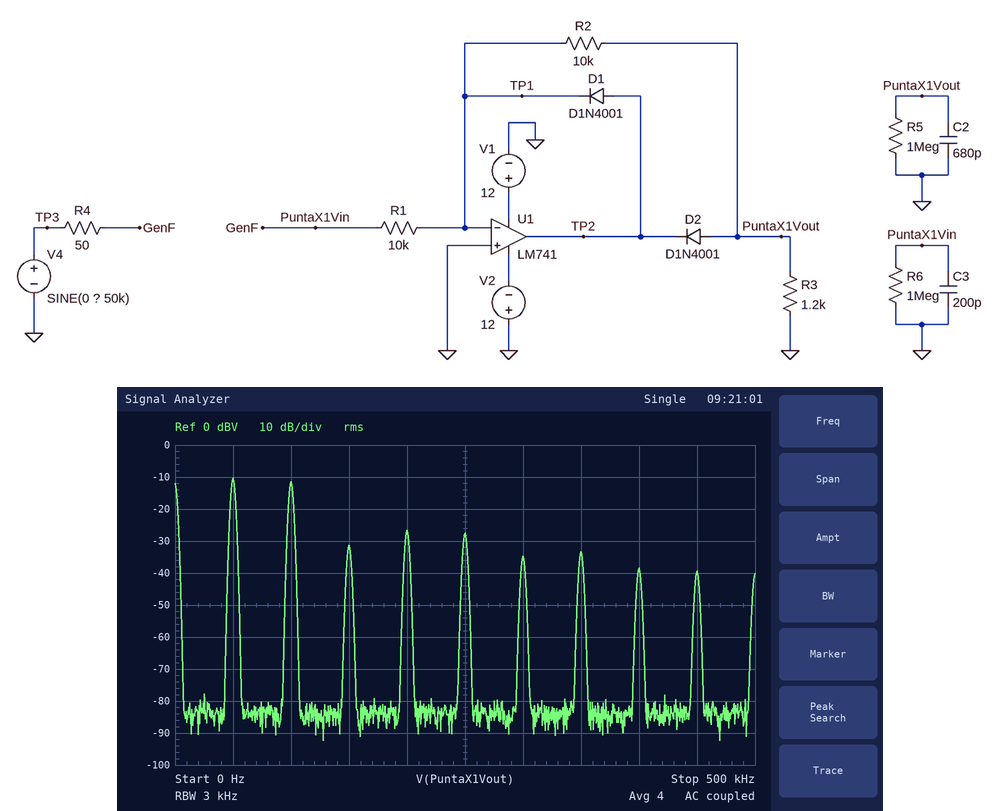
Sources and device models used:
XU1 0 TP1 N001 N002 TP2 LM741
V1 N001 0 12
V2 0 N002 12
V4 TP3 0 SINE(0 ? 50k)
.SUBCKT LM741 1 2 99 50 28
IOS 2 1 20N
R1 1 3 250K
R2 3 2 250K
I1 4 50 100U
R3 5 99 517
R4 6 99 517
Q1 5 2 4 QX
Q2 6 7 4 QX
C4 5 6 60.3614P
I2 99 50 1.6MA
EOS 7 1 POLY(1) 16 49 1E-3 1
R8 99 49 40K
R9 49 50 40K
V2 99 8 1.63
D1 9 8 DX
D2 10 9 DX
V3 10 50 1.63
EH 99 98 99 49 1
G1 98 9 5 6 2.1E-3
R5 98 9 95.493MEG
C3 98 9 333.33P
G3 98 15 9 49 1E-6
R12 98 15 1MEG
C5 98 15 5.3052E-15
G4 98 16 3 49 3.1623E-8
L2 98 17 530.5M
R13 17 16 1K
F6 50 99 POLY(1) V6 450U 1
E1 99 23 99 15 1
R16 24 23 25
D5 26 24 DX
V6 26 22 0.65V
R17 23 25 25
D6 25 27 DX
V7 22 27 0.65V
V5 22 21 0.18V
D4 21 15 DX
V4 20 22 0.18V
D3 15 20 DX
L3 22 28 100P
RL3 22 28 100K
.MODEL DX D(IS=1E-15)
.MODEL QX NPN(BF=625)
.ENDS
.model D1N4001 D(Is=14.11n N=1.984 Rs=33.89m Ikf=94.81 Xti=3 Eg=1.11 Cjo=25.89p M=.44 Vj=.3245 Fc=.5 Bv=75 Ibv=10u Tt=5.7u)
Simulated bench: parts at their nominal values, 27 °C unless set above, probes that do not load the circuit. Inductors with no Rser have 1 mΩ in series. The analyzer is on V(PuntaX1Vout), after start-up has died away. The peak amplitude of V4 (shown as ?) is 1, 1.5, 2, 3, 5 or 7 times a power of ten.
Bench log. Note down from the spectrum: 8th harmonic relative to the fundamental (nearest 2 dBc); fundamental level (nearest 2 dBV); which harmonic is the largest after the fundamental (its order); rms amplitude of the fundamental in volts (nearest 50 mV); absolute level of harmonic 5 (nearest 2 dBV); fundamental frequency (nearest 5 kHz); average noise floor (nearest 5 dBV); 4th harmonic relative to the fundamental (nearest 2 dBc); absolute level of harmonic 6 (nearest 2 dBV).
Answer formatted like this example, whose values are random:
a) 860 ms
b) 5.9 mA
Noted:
a) -28 dBc
b) -10 dBV
c) 2
d) 300 mV
e) -28 dBV
f) 50 kHz
g) -85 dBV
h) -16 dBc
i) -34 dBV
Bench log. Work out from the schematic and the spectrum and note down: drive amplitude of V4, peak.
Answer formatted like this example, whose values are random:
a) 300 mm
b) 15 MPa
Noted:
a) 7 V
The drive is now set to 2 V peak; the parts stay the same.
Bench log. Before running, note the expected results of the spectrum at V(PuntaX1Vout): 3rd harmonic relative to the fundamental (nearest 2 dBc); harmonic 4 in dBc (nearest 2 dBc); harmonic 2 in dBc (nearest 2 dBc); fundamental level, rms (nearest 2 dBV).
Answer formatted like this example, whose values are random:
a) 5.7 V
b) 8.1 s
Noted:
a) -6 dBc
b) -28 dBc
c) 0 dBc
d) -14 dBV
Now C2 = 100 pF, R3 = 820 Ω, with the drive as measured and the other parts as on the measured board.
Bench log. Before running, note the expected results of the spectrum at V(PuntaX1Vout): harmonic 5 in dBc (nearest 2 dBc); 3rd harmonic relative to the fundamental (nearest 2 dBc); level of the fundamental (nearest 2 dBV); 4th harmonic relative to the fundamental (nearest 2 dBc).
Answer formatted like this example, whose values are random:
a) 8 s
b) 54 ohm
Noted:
a) -14 dBc
b) -22 dBc
c) -10 dBV
d) -14 dBc
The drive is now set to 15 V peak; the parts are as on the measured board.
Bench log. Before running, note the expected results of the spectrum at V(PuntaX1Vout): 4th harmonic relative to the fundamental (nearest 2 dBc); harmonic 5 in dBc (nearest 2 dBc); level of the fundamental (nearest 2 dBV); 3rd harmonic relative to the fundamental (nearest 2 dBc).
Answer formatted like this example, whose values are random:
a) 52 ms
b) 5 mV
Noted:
a) -18 dBc
b) -16 dBc
c) -10 dBV
d) -24 dBc
